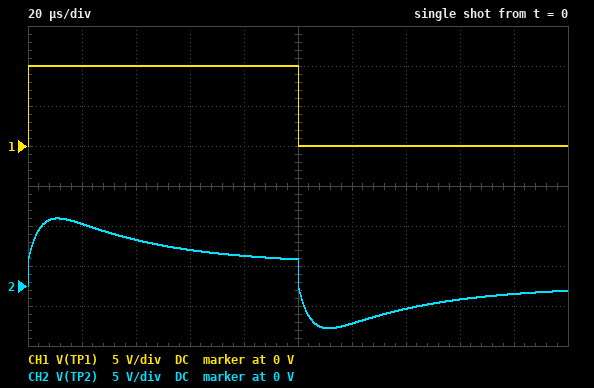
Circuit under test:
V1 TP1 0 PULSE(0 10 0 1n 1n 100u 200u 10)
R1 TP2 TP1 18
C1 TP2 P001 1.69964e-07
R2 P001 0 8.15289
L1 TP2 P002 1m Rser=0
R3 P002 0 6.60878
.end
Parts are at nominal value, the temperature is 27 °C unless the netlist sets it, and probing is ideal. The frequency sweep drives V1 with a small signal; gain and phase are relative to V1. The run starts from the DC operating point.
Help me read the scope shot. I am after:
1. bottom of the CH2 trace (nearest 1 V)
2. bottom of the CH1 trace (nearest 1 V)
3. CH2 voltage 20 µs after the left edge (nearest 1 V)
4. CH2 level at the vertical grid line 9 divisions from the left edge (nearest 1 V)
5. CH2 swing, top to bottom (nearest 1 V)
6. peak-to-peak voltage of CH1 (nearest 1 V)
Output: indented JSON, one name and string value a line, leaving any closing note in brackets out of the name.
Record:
{
  "bottom of the CH2 trace": "-5 V",
  "bottom of the CH1 trace": "0 V",
  "CH2 voltage 20 µs after the left edge": "8 V",
  "CH2 level at the vertical grid line 9 divisions from the left edge": "-1 V",
  "CH2 swing, top to bottom": "14 V",
  "peak-to-peak voltage of CH1": "10 V"
}
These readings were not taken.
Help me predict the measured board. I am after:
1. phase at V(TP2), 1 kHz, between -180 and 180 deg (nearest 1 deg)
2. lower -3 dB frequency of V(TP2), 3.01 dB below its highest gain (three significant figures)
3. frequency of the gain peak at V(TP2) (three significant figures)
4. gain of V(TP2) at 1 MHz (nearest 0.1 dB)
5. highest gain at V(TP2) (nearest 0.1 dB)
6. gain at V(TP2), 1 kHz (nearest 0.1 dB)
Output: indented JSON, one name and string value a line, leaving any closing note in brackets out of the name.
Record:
{
  "phase at V(TP2), 1 kHz, between -180 and 180 deg": "29 deg",
  "lower -3 dB frequency of V(TP2), 3.01 dB below its highest gain": "3.17 kHz",
  "frequency of the gain peak at V(TP2)": "11.9 kHz",
  "gain of V(TP2) at 1 MHz": "-10.1 dB",
  "highest gain at V(TP2)": "-0.4 dB",
  "gain at V(TP2), 1 kHz": "-8.9 dB"
}
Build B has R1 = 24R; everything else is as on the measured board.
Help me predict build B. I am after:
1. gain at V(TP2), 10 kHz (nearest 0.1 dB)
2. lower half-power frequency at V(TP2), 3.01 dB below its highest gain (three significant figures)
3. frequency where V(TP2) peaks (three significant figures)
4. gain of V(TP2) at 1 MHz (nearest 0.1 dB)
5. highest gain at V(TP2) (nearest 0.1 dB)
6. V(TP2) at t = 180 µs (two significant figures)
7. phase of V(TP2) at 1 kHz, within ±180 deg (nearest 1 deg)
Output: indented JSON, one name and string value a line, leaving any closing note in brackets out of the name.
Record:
{
  "gain at V(TP2), 10 kHz": "-0.6 dB",
  "lower half-power frequency at V(TP2), 3.01 dB below its highest gain": "3.87 kHz",
  "frequency where V(TP2) peaks": "12.0 kHz",
  "gain of V(TP2) at 1 MHz": "-11.9 dB",
  "highest gain at V(TP2)": "-0.5 dB",
  "V(TP2) at t = 180 µs": "-670 mV",
  "phase of V(TP2) at 1 kHz, within ±180 deg": "32 deg"
}
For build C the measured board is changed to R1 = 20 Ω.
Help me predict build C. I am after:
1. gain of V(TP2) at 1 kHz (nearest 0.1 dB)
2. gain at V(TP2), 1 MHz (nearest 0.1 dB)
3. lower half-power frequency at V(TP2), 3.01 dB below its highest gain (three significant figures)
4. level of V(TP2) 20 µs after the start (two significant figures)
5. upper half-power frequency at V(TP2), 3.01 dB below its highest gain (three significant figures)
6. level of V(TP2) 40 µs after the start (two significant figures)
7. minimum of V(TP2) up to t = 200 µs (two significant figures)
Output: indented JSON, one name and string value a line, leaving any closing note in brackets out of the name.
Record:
{
  "gain of V(TP2) at 1 kHz": "-9.5 dB",
  "gain at V(TP2), 1 MHz": "-10.7 dB",
  "lower half-power frequency at V(TP2), 3.01 dB below its highest gain": "3.42 kHz",
  "level of V(TP2) 20 µs after the start": "7.6 V",
  "upper half-power frequency at V(TP2), 3.01 dB below its highest gain": "42.4 kHz",
  "level of V(TP2) 40 µs after the start": "5.5 V",
  "minimum of V(TP2) up to t = 200 µs": "-5.4 V"
}
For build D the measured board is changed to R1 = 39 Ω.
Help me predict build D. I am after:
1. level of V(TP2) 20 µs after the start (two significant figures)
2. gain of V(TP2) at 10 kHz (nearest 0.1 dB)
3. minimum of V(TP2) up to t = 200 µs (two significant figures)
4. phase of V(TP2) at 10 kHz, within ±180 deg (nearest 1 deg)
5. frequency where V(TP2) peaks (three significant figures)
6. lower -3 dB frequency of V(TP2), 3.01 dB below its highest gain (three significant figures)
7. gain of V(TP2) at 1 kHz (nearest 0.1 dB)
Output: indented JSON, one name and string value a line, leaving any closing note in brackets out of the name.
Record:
{
  "level of V(TP2) 20 µs after the start": "6.4 V",
  "gain of V(TP2) at 10 kHz": "-1.0 dB",
  "minimum of V(TP2) up to t = 200 µs": "-5.5 V",
  "phase of V(TP2) at 10 kHz, within ±180 deg": "10 deg",
  "frequency where V(TP2) peaks": "12.0 kHz",
  "lower -3 dB frequency of V(TP2), 3.01 dB below its highest gain": "5.20 kHz",
  "gain of V(TP2) at 1 kHz": "-14.0 dB"
}
